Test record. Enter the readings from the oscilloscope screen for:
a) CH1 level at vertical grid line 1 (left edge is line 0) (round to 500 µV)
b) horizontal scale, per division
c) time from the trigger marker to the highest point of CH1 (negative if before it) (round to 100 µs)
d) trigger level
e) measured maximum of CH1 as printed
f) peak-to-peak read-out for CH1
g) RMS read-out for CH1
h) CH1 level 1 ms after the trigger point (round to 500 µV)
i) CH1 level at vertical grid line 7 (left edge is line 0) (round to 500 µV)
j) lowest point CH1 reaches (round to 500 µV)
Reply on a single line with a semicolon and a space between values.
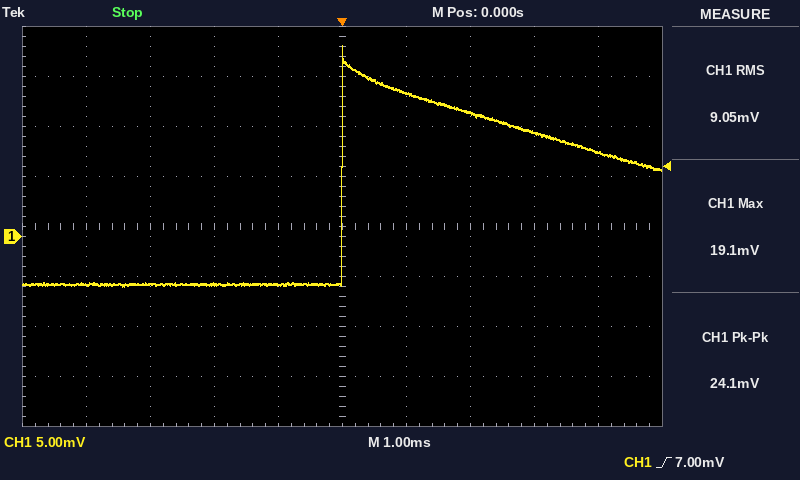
-5.0 mV; 1 ms; 0.0 ms; 7.00 mV; 19.1 mV; 24.1 mV; 9.05 mV; 14.5 mV; 12.5 mV; -5.0 mV
